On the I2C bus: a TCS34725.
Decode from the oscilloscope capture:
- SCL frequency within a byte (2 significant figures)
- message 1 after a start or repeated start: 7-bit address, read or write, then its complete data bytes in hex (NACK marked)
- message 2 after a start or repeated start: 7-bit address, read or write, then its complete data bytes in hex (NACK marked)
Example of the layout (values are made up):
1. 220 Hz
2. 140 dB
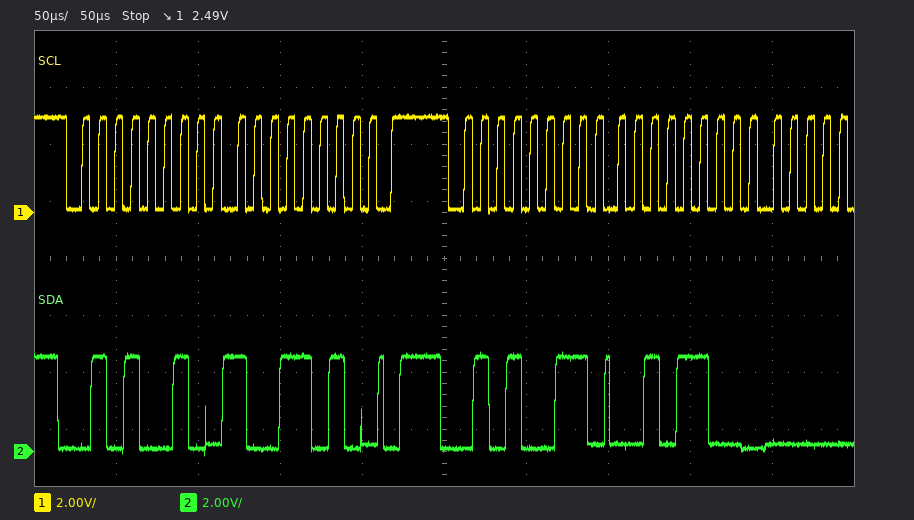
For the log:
1. 100 kHz
2. 0x29 write: 9A
3. 0x29 read: 2C
